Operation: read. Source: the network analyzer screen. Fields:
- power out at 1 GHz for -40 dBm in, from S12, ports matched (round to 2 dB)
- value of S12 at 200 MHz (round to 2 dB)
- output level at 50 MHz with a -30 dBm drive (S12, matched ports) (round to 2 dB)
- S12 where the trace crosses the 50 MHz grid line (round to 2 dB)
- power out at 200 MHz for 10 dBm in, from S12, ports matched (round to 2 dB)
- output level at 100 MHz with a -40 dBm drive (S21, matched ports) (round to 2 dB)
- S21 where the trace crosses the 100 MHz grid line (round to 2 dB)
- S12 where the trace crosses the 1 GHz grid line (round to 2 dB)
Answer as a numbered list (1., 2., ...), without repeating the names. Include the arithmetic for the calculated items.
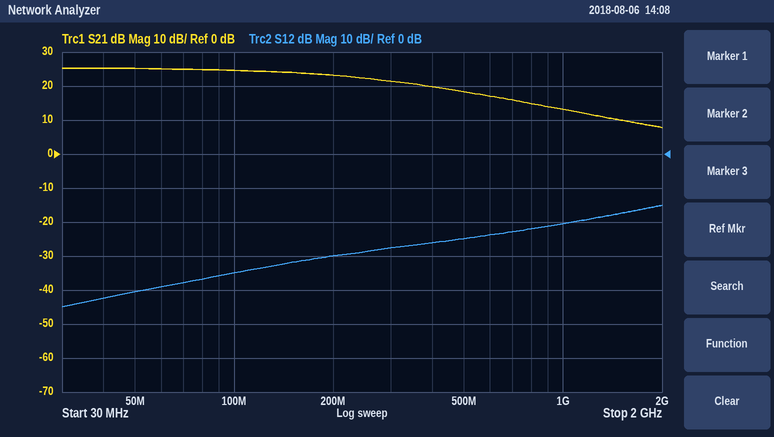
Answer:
1. -40 dBm + (-20 dB) = -60 dBm
2. -30 dB
3. -30 dBm + (-40 dB) = -70 dBm
4. -40 dB
5. 10 dBm + (-30 dB) = -20 dBm
6. -40 dBm + (24 dB) = -16 dBm
7. 24 dB
8. -20 dB
